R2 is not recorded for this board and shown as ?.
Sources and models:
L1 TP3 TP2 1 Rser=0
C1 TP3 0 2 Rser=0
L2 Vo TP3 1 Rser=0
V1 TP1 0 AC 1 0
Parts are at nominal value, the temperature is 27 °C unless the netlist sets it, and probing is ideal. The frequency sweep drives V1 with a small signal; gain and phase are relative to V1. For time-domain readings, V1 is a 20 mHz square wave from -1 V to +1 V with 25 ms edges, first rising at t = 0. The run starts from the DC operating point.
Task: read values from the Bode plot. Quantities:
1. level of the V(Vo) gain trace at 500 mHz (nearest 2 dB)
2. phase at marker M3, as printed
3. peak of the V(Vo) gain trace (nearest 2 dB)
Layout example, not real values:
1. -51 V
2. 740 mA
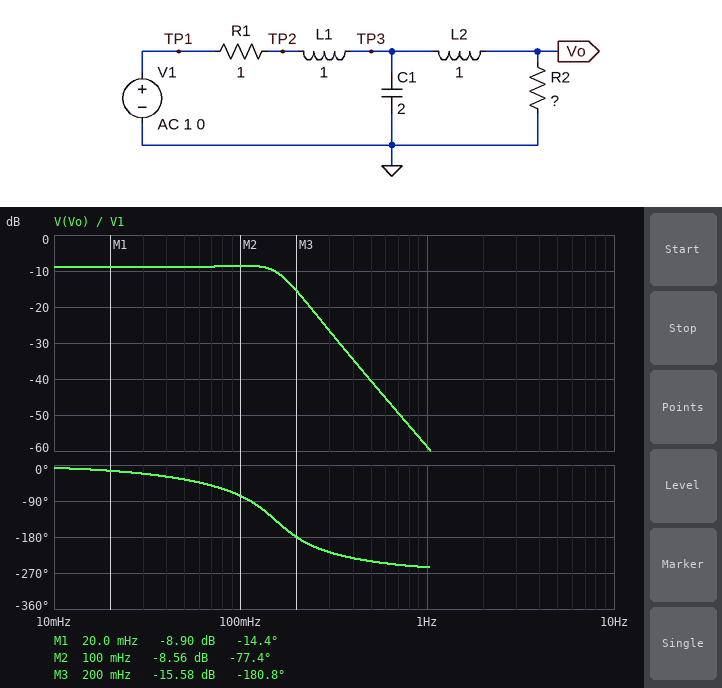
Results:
1. -40 dB
2. -180.8 deg
3. -8 dB
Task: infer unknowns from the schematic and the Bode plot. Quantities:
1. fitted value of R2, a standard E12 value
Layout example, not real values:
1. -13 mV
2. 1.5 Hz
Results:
1. 0.56 Ω
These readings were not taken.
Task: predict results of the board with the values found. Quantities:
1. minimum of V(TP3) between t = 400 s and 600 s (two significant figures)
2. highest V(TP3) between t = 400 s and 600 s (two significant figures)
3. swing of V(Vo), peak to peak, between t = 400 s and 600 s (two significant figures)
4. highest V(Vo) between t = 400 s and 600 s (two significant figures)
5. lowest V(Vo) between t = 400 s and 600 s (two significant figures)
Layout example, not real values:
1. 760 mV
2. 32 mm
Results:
1. -680 mV
2. 680 mV
3. 900 mV
4. 450 mV
5. -450 mV
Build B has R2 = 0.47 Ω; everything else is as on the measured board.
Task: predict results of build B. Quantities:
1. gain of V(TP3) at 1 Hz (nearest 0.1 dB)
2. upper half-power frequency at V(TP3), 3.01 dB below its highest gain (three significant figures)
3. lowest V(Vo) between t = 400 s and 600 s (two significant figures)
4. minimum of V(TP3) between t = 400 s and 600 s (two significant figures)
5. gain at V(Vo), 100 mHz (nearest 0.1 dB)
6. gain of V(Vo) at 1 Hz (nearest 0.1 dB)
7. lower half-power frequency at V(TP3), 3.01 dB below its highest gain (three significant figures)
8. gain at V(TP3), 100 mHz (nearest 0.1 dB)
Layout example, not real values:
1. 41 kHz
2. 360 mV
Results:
1. -37.8 dB
2. 188 mHz
3. -410 mV
4. -690 mV
5. -9.4 dB
6. -60.4 dB
7. 79.5 mHz
8. -4.9 dB
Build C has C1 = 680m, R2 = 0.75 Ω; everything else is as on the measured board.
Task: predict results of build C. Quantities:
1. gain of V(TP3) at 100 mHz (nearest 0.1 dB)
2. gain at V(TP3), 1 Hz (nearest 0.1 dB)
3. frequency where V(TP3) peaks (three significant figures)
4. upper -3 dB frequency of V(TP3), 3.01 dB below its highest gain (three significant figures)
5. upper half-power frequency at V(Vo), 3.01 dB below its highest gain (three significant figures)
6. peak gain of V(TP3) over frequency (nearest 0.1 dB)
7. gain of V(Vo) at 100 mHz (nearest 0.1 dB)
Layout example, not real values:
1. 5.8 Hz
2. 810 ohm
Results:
1. -5.8 dB
2. -28.0 dB
3. 255 mHz
4. 319 mHz
5. 299 mHz
6. -0.1 dB
7. -8.1 dB
